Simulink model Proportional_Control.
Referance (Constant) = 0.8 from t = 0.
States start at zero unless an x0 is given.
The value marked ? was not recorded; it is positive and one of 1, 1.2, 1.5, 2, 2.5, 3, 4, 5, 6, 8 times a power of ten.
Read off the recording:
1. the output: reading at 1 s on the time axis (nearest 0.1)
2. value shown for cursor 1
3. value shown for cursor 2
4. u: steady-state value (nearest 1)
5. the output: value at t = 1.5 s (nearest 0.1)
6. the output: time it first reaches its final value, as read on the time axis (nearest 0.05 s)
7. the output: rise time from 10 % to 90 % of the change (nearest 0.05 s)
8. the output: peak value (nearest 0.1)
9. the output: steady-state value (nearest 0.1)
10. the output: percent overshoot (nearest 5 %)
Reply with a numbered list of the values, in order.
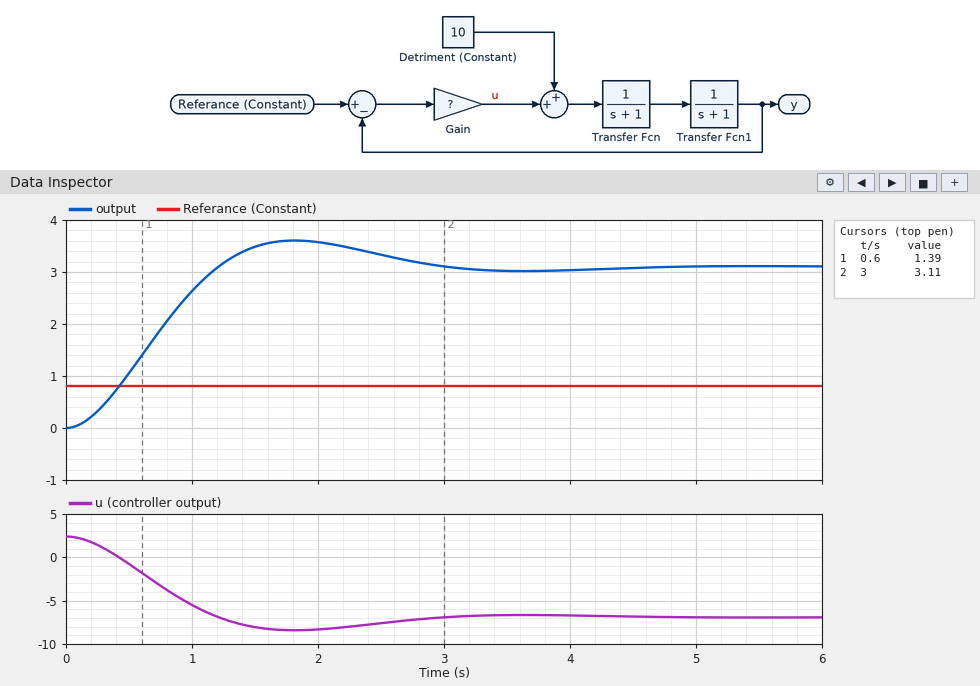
1. 2.6
2. 1.39
3. 3.11
4. -7
5. 3.5
6. 1.20 s
7. 0.80 s
8. 3.6
9. 3.1
10. 15 %
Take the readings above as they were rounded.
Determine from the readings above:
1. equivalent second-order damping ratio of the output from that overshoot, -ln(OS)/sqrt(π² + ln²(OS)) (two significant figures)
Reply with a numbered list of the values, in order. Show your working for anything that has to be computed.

1. ln(0.15) = -1.897; 1.897 / sqrt(9.870 + 3.599) = 0.52
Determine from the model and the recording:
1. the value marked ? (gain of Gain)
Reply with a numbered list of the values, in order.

1. 3
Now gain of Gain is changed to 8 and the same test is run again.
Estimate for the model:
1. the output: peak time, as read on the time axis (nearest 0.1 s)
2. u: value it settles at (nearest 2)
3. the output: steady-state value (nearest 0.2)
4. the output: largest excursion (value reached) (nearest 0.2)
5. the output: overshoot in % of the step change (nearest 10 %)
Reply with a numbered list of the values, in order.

1. 1.1 s
2. -8
3. 1.8
4. 2.4
5. 30 %
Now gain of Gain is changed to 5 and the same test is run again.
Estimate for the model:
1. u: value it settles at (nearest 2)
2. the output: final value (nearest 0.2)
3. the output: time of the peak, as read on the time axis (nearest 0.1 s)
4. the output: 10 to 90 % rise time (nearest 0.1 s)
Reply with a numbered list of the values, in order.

1. -8
2. 2.4
3. 1.4 s
4. 0.6 s
